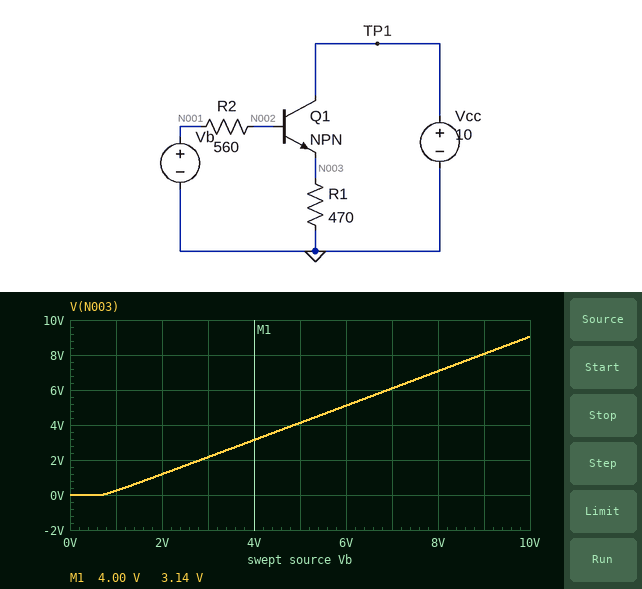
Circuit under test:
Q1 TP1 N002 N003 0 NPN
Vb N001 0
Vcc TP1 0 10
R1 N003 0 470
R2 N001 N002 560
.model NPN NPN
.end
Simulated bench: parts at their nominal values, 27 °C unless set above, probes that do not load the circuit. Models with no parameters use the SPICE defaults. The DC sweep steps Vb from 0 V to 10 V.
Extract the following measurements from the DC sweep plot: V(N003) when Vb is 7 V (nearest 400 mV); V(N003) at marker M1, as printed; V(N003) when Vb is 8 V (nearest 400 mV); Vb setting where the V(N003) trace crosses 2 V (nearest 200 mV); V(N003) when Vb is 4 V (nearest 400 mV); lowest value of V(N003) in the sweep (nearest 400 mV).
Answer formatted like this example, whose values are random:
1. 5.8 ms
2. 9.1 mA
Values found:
1. 6.0 V
2. 3.14 V
3. 7.2 V
4. 2.8 V
5. 3.2 V
6. 0 V
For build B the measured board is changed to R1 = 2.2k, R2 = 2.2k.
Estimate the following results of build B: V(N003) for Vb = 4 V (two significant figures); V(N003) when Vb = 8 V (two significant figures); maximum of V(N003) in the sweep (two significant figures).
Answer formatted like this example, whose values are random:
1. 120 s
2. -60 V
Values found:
1. 3.2 V
2. 7.1 V
3. 9.1 V
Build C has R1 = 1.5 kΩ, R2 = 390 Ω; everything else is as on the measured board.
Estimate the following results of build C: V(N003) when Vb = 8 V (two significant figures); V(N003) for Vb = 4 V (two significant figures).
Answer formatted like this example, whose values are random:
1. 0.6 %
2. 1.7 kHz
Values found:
1. 7.2 V
2. 3.2 V
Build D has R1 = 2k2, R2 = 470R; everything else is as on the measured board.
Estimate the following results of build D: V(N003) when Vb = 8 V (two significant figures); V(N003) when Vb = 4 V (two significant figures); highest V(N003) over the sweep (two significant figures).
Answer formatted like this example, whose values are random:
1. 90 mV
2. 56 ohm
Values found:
1. 7.2 V
2. 3.2 V
3. 9.2 V
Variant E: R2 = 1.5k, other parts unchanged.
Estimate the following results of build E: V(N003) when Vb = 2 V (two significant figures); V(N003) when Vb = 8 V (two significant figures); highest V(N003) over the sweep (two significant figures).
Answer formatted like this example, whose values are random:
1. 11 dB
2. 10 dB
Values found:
1. 1.2 V
2. 6.9 V
3. 8.9 V
